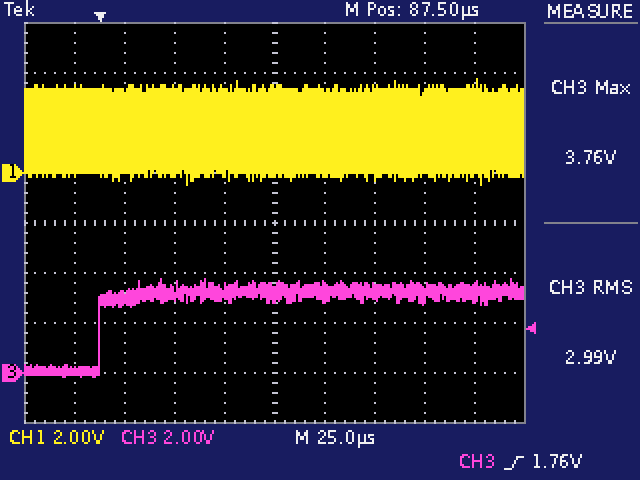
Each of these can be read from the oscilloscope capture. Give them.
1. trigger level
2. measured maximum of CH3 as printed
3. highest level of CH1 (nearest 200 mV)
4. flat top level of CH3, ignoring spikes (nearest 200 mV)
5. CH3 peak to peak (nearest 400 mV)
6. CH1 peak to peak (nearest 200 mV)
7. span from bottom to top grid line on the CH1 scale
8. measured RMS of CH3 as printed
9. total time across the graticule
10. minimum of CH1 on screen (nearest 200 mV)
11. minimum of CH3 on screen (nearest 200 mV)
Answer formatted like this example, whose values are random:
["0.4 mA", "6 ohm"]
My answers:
["1.76 V", "3.76 V", "3.8 V", "3.2 V", "4.0 V", "4.2 V", "16 V", "2.99 V", "250 µs", "-400 mV", "-200 mV"]
